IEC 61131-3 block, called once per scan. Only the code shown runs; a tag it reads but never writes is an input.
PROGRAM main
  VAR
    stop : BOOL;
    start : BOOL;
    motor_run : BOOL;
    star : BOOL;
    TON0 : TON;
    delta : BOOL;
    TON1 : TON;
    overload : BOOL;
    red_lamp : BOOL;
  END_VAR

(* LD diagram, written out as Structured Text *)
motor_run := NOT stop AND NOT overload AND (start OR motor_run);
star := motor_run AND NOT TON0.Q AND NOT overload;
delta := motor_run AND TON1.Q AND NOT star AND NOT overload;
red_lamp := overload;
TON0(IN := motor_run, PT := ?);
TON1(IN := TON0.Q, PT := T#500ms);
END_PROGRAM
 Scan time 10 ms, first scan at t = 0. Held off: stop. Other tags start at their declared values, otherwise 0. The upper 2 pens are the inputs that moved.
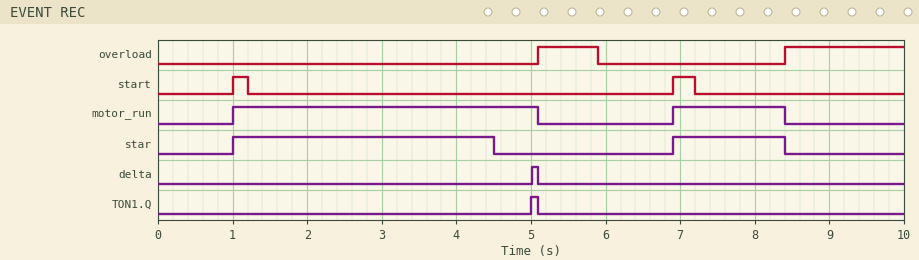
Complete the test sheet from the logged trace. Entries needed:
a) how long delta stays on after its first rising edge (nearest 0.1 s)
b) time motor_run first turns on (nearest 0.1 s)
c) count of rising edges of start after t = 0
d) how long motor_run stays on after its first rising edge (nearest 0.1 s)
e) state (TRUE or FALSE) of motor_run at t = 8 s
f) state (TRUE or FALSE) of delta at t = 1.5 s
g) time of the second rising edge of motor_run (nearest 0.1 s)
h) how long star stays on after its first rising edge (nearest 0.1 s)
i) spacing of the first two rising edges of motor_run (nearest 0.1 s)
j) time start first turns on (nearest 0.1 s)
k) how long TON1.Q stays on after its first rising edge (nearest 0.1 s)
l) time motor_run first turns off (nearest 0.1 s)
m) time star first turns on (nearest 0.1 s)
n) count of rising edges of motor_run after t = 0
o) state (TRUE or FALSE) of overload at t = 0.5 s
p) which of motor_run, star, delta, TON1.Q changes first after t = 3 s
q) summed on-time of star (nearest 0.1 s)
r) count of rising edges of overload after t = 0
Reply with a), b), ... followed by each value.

a) 0.1 s
b) 1.0 s
c) 2
d) 4.1 s
e) TRUE
f) FALSE
g) 6.9 s
h) 3.5 s
i) 5.9 s
j) 1.0 s
k) 0.1 s
l) 5.1 s
m) 1.0 s
n) 2
o) FALSE
p) star
q) 5.0 s
r) 2
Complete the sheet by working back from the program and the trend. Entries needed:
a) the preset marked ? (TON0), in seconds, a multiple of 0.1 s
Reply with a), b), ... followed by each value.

a) 3.5 s
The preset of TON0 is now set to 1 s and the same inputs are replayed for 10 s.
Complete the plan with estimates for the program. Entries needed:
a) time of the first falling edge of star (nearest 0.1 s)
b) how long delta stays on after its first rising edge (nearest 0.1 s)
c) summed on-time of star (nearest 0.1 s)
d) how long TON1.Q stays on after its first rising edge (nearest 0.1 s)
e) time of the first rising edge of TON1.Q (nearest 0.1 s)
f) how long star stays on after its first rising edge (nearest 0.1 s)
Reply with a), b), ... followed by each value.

a) 2.0 s
b) 2.6 s
c) 2.0 s
d) 2.6 s
e) 2.5 s
f) 1.0 s
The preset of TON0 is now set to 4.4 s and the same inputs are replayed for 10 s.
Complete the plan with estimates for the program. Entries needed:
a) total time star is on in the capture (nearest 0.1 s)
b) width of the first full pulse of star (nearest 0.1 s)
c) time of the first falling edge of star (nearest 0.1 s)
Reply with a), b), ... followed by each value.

a) 5.6 s
b) 4.1 s
c) 5.1 s
